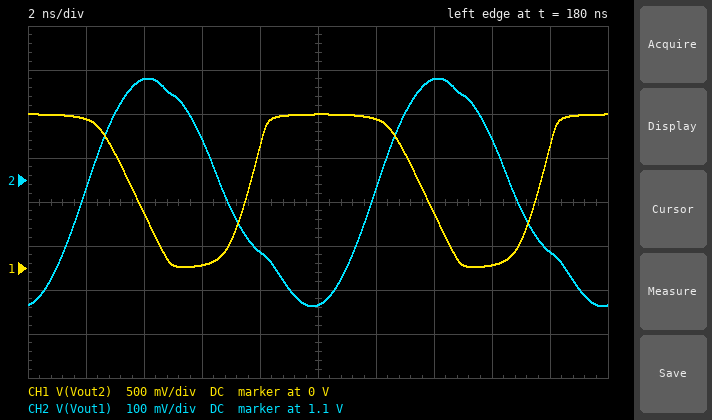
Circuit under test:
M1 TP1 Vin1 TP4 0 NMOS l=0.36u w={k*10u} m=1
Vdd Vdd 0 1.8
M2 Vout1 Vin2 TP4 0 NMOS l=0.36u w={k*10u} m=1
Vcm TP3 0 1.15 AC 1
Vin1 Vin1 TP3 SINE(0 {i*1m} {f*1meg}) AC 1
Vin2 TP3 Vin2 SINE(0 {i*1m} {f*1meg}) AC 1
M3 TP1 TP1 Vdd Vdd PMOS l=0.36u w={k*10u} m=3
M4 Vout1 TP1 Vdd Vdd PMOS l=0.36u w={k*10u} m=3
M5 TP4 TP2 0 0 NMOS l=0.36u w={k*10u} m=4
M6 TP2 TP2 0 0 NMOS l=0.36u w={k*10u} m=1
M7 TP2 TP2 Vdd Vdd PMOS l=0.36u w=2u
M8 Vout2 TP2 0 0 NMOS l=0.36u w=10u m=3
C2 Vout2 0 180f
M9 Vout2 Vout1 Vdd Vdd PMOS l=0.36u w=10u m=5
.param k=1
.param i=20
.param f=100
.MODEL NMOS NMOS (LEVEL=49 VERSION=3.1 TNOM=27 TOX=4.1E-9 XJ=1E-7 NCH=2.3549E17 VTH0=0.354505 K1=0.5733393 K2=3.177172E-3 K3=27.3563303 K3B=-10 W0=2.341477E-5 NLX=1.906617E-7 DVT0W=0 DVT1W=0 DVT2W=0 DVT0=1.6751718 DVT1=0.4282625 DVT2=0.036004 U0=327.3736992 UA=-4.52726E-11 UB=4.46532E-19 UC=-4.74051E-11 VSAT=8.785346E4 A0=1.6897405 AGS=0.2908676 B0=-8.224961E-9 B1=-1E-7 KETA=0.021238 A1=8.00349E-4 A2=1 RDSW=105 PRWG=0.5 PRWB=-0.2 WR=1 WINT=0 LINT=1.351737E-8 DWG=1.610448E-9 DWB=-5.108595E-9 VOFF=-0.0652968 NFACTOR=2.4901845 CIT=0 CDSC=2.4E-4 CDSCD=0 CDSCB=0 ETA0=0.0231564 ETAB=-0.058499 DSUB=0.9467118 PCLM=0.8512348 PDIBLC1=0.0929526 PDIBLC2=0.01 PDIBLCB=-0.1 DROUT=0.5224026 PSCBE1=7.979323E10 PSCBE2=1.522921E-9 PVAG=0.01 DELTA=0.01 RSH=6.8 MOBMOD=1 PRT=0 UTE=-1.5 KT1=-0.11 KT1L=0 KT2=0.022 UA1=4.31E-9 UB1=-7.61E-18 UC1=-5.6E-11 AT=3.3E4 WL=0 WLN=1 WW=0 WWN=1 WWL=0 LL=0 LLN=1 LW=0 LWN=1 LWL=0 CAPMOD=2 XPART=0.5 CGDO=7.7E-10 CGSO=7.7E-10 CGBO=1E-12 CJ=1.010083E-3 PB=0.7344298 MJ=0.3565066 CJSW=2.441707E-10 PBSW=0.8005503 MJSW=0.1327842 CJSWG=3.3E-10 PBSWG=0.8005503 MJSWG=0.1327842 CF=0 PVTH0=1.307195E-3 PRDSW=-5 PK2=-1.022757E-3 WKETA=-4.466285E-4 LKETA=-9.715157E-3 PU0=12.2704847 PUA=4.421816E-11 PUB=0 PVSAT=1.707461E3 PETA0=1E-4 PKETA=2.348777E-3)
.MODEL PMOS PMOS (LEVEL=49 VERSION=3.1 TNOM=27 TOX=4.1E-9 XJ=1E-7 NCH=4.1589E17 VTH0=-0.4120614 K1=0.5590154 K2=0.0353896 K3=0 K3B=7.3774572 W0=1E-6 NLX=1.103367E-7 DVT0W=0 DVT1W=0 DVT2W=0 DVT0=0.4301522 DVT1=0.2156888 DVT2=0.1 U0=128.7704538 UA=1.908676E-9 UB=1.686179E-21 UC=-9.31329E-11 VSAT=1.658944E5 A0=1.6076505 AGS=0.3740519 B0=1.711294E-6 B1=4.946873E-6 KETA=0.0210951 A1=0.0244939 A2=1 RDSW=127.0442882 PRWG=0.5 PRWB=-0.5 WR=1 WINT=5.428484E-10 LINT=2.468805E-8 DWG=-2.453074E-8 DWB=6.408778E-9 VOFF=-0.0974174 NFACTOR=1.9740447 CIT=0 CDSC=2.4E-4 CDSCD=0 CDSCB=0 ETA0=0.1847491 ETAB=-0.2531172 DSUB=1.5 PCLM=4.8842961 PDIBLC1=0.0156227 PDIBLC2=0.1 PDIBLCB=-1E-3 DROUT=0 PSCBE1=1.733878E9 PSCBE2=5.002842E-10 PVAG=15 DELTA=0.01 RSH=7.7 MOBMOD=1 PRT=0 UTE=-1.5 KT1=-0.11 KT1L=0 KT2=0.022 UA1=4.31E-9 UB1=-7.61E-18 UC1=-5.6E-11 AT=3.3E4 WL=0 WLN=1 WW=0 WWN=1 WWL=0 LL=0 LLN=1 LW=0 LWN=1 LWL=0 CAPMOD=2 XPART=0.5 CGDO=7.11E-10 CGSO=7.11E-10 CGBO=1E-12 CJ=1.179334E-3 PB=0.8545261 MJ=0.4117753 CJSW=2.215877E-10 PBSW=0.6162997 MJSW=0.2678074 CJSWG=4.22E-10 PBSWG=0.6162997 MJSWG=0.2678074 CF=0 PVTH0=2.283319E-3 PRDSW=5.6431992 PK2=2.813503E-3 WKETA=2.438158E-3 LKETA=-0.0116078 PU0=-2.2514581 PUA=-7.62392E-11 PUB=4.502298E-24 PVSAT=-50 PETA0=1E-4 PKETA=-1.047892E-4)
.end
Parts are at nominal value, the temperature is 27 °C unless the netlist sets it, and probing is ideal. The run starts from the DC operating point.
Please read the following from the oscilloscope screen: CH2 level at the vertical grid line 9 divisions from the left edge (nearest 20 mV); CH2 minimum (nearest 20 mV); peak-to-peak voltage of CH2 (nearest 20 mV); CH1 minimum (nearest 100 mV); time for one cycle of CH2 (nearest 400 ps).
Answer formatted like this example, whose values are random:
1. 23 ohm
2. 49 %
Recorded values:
1. 940 mV
2. 820 mV
3. 520 mV
4. 0 V
5. 10.0 ns
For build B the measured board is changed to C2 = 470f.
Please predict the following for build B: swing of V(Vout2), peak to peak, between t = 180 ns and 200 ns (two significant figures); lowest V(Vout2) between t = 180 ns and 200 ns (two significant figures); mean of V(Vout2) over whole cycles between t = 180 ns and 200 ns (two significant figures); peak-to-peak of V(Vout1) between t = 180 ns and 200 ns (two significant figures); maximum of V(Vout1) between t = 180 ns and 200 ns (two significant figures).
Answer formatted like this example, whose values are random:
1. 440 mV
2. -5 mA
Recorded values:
1. 1.5 V
2. 250 mV
3. 1.2 V
4. 620 mV
5. 1.4 V
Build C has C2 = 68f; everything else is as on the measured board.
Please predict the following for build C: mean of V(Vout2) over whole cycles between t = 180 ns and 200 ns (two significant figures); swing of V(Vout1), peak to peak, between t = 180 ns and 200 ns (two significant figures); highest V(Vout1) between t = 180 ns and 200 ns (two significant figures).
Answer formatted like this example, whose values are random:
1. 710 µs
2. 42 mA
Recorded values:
1. 1.0 V
2. 470 mV
3. 1.3 V
